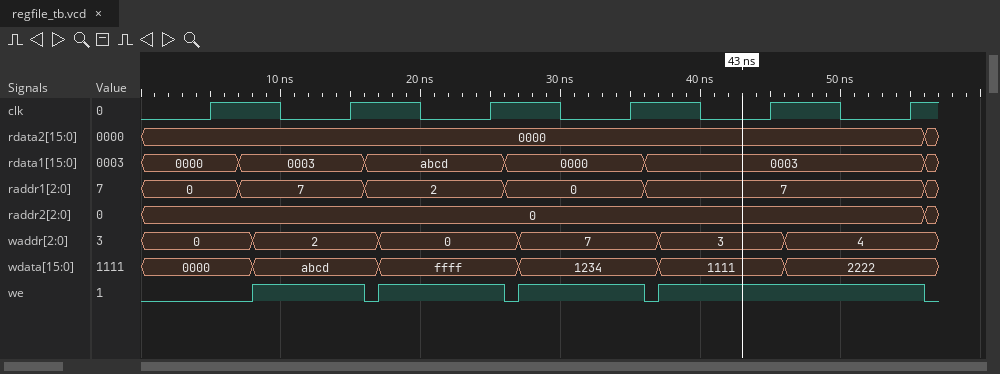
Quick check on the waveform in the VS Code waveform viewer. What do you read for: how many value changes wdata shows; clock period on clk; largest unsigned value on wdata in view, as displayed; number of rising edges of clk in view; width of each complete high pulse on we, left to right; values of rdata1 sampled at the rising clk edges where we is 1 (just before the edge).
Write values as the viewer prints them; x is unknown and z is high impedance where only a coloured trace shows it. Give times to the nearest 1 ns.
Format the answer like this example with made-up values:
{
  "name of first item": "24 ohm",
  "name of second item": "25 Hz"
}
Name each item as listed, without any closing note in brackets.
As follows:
{
  "how many value changes wdata shows": "5",
  "clock period on clk": "10 ns",
  "largest unsigned value on wdata in view, as displayed": "ffff",
  "number of rising edges of clk in view": "6",
  "width of each complete high pulse on we, left to right": "8 ns, 9 ns, 9 ns, 19 ns",
  "values of rdata1 sampled at the rising clk edges where we is 1": "0003, abcd, 0000, 0003, 0003"
}
